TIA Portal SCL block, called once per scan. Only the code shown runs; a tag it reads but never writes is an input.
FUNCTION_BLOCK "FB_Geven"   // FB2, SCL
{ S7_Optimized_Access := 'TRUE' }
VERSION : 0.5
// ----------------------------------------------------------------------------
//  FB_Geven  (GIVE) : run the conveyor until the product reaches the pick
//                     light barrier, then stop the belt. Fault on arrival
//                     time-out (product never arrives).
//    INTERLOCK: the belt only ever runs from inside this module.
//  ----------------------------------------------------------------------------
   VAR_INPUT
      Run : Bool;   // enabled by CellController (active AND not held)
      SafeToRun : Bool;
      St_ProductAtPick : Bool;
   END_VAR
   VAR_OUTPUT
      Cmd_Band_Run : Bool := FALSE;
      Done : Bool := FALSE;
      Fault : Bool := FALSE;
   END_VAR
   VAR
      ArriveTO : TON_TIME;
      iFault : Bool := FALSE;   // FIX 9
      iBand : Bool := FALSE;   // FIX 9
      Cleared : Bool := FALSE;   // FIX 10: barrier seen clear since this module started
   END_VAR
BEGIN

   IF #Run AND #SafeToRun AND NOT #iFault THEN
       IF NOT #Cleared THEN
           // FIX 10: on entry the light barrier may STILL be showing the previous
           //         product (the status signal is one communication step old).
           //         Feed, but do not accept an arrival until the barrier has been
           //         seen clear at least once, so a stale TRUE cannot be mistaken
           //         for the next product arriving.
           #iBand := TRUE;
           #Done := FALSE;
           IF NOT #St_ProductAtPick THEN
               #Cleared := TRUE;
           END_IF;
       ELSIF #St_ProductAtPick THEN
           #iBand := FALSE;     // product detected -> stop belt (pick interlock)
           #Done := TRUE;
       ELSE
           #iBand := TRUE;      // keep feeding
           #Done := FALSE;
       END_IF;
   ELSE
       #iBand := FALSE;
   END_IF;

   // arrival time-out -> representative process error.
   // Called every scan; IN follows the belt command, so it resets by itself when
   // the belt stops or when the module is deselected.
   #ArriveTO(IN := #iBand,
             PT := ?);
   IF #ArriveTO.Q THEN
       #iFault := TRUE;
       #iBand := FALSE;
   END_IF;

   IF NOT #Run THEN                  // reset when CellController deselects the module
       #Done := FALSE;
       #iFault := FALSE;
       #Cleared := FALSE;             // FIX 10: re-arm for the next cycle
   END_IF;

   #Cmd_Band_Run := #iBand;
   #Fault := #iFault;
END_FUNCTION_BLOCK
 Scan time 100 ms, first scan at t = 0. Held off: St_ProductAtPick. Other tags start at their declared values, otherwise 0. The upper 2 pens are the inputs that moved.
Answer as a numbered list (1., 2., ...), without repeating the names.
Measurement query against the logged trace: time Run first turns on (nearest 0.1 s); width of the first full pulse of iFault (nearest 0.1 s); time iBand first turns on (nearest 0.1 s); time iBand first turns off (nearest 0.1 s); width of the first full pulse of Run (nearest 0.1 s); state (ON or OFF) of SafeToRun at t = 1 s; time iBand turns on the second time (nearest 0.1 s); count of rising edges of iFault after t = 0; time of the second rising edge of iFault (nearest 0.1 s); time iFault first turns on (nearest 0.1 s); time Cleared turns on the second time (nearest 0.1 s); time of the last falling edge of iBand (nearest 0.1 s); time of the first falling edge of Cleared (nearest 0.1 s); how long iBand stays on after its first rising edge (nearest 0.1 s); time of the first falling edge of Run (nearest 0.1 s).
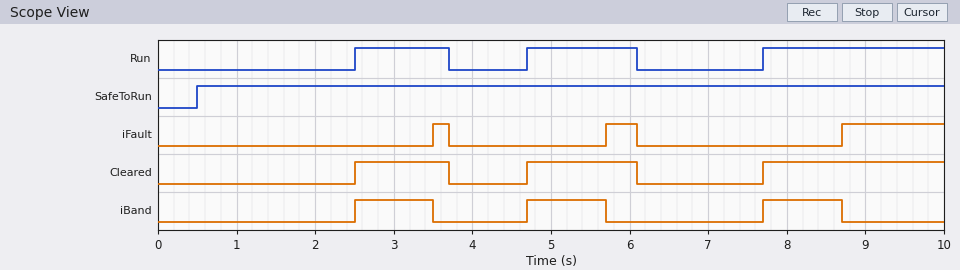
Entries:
1. 2.5 s
2. 0.2 s
3. 2.5 s
4. 3.5 s
5. 1.2 s
6. ON
7. 4.7 s
8. 3
9. 5.7 s
10. 3.5 s
11. 4.7 s
12. 8.7 s
13. 3.7 s
14. 1.0 s
15. 3.7 s
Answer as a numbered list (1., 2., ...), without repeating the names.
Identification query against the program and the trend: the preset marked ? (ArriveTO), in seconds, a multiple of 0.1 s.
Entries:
1. 1.0 s
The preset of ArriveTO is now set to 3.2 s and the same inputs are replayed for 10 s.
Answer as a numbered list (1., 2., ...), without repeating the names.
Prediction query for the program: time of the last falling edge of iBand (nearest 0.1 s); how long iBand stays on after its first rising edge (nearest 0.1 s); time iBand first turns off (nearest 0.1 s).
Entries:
1. 6.1 s
2. 1.2 s
3. 3.7 s
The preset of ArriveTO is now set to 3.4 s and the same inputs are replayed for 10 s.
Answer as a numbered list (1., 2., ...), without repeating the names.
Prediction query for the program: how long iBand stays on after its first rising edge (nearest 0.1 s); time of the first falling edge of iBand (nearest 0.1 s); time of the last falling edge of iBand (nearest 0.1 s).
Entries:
1. 1.2 s
2. 3.7 s
3. 6.1 s
